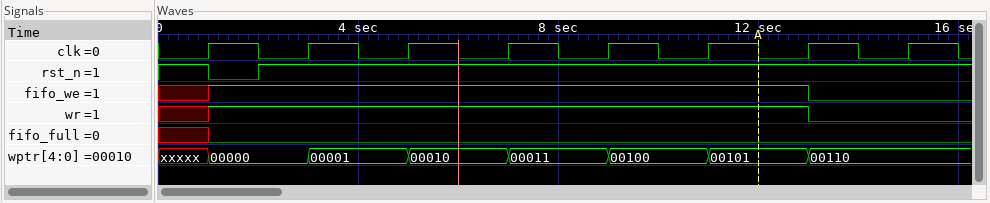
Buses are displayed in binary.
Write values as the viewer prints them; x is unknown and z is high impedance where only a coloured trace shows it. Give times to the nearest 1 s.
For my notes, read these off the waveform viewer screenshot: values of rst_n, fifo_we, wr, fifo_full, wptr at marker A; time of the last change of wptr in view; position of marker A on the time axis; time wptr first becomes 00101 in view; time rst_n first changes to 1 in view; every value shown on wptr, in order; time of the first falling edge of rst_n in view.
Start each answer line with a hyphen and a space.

- rst_n=1, fifo_we=1, wr=1, fifo_full=0, wptr=00101
- 13 s
- 12 s
- 11 s
- 2 s
- xxxxx, 00000, 00001, 00010, 00011, 00100, 00101, 00110
- 1 s
